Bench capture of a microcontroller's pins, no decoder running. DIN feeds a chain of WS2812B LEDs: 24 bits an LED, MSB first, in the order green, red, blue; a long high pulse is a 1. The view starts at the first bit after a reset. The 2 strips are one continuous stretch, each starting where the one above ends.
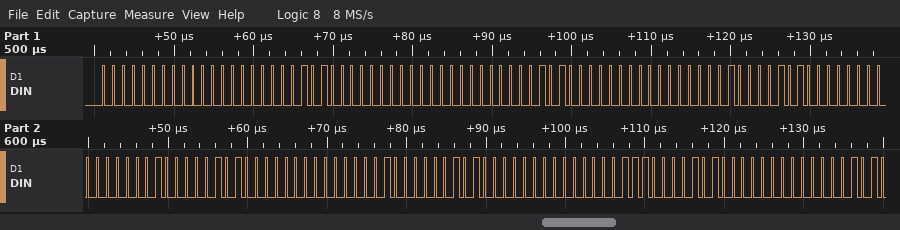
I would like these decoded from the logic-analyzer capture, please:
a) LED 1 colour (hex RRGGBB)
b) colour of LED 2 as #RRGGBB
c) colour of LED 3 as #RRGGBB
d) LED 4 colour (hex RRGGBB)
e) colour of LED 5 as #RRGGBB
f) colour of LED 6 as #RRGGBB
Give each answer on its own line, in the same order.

#00000A
#00000A
#01000A
#02000A
#04000A
#07000A
